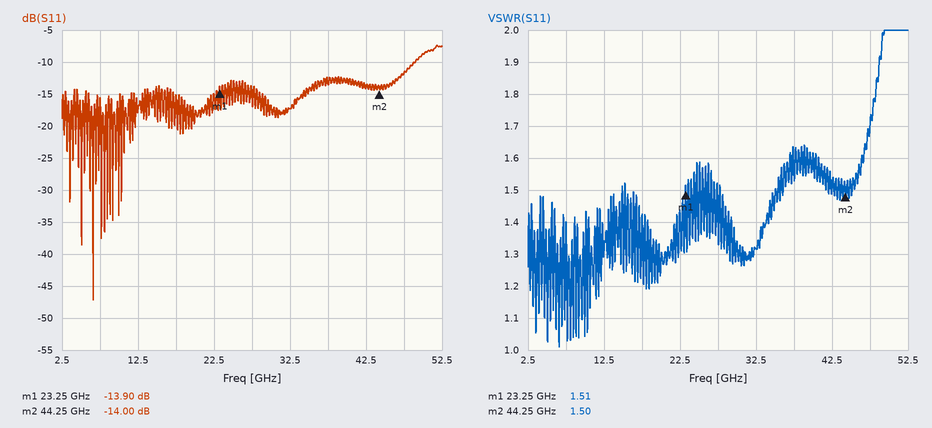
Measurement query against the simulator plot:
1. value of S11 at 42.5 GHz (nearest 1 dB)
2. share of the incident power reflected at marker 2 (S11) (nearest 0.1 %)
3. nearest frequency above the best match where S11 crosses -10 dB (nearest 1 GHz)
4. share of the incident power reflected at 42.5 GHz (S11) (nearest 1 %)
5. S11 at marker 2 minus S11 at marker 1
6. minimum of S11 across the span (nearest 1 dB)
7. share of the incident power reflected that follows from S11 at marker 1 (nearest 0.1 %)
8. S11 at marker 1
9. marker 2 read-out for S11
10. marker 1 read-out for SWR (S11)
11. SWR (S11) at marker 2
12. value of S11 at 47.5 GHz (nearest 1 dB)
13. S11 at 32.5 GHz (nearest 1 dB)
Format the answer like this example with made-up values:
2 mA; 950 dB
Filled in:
-14 dB; 4.0 %; 49 GHz; 4 %; -0.10 dB; -47 dB; 4.1 %; -13.90 dB; -14.00 dB; 1.51; 1.50; -12 dB; -17 dB
